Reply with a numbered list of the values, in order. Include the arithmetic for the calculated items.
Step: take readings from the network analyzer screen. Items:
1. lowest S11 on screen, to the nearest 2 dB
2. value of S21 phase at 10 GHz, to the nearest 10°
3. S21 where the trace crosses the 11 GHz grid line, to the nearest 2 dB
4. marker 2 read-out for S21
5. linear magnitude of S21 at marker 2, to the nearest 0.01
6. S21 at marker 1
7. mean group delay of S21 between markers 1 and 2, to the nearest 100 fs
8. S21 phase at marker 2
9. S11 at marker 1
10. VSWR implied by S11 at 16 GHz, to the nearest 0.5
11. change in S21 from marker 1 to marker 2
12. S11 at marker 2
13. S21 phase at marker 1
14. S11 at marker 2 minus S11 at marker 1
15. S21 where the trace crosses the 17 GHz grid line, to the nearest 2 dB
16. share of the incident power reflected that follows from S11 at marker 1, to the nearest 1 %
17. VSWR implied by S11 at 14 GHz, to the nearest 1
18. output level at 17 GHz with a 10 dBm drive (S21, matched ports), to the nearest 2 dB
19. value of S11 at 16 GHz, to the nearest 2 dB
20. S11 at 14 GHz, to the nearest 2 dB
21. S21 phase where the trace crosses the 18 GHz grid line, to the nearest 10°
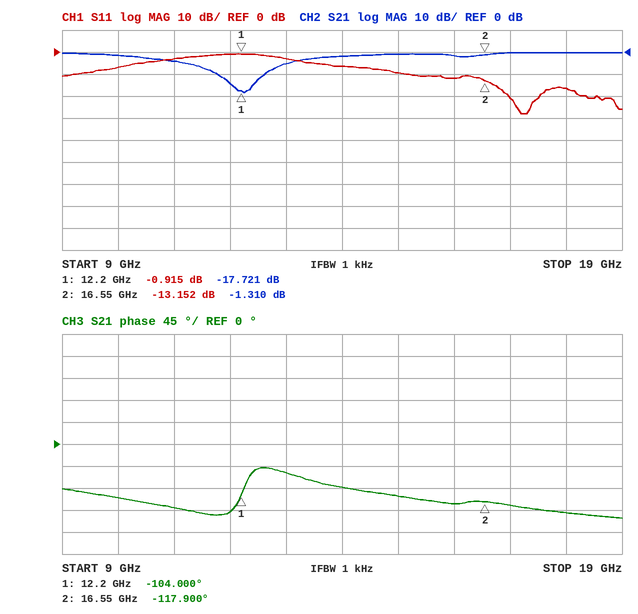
1. -28 dB
2. -110°
3. -4 dB
4. -1.310 dB
5. 10^(-1.31/20) ≈ 0.86
6. -17.721 dB
7. −(-117.9° − (-104°))/(360° × 4.35 GHz) ≈ 8.9 ps
8. -117.900°
9. -0.915 dB
10. |Γ| = 10^(-12/20) = 0.2512; VSWR = (1 + 0.2512)/(1 − 0.2512) ≈ 1.67, so 1.5 to the nearest 0.5
11. -1.31 − (-17.721) = 16.411 dB
12. -13.152 dB
13. -104.000°
14. -13.152 − (-0.915) = -12.237 dB
15. 0 dB
16. 10^(-0.915/10) ≈ 81 %
17. |Γ| = 10^(-6/20) = 0.5012; VSWR = (1 + 0.5012)/(1 − 0.5012) ≈ 3
18. 10 dBm + (0 dB) = 10 dBm
19. -12 dB
20. -6 dB
21. -140°
